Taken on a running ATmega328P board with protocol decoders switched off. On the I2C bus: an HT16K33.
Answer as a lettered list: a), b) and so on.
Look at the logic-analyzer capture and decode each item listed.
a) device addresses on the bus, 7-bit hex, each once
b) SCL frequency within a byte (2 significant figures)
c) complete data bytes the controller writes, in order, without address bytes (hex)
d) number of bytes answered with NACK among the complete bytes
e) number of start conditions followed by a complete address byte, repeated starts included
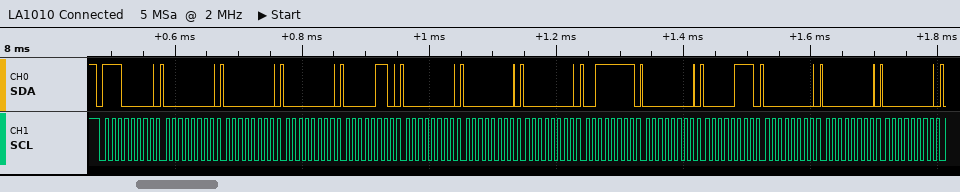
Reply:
a) 0x70
b) 100 kHz
c) 00 00 00 06 00 00 00 3F 00 07 00 00 00
d) 0
e) 1
